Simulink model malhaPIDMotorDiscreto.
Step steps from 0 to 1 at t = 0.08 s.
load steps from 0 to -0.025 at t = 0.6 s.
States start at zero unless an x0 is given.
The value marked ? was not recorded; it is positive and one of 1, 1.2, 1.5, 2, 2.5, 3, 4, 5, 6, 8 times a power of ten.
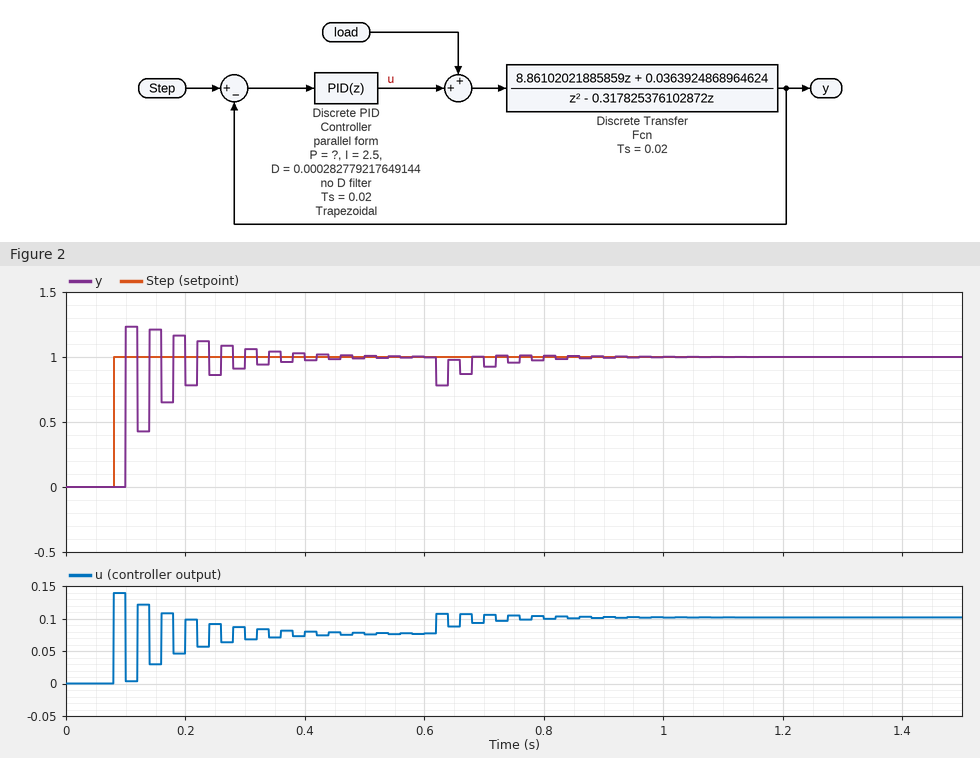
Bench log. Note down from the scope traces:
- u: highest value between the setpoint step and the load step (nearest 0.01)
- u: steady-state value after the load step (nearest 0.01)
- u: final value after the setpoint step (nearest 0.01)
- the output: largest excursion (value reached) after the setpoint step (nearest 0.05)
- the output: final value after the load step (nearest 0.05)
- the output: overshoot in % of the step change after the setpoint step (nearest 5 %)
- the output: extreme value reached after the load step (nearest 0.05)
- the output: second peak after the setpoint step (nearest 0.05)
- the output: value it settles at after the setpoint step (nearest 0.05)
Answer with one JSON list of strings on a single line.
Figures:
["0.14", "0.10", "0.08", "1.25", "1.00", "25 %", "0.80", "1.20", "1.00"]
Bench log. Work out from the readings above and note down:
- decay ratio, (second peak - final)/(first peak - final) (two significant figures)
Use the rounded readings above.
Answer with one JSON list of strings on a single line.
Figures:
["0.80"]
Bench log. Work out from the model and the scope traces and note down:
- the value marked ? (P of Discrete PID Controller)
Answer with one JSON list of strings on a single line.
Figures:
["0.1"]
